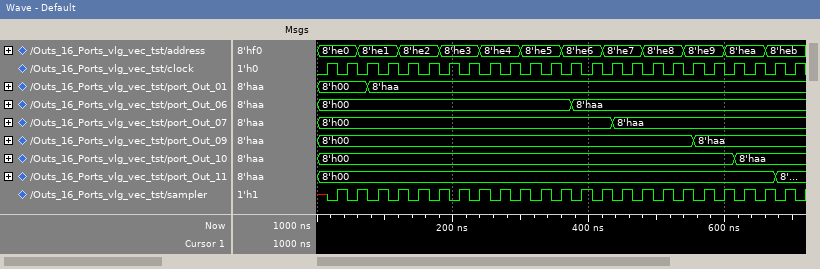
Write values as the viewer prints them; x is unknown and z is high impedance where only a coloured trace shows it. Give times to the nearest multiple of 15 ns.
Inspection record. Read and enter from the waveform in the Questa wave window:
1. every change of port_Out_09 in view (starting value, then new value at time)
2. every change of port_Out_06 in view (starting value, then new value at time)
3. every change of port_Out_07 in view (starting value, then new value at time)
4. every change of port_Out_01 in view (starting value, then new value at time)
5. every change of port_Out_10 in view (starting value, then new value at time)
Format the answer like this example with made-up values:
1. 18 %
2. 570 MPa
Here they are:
1. 8'h00, 8'haa at 555 ns
2. 8'h00, 8'haa at 375 ns
3. 8'h00, 8'haa at 435 ns
4. 8'h00, 8'haa at 75 ns
5. 8'h00, 8'haa at 615 ns
